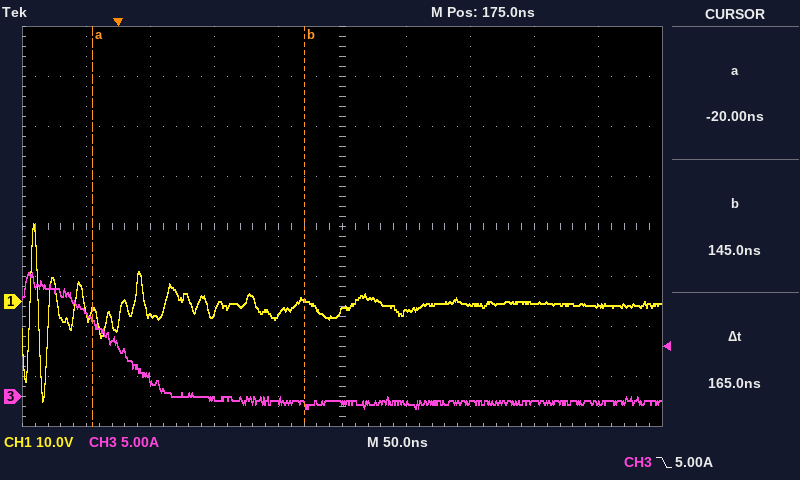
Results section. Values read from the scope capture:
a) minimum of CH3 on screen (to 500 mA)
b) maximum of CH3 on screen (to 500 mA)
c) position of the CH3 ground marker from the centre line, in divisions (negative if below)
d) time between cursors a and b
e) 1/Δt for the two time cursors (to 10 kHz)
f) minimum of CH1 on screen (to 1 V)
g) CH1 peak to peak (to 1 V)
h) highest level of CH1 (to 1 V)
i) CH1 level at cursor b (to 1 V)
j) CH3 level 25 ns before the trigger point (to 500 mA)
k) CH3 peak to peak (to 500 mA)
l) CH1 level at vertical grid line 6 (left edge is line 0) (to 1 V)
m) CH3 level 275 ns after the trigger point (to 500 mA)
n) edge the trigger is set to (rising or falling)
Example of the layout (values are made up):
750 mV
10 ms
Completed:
-1.0 A
12.5 A
-3.4 div
165 ns
6.06 MHz
-20 V
36 V
16 V
0 V
8.5 A
13.5 A
-2 V
-500 mA
falling
